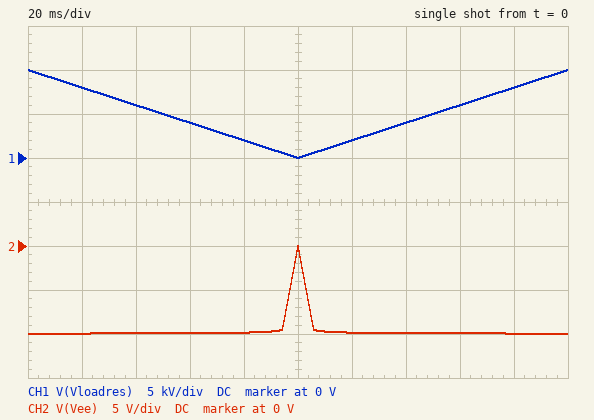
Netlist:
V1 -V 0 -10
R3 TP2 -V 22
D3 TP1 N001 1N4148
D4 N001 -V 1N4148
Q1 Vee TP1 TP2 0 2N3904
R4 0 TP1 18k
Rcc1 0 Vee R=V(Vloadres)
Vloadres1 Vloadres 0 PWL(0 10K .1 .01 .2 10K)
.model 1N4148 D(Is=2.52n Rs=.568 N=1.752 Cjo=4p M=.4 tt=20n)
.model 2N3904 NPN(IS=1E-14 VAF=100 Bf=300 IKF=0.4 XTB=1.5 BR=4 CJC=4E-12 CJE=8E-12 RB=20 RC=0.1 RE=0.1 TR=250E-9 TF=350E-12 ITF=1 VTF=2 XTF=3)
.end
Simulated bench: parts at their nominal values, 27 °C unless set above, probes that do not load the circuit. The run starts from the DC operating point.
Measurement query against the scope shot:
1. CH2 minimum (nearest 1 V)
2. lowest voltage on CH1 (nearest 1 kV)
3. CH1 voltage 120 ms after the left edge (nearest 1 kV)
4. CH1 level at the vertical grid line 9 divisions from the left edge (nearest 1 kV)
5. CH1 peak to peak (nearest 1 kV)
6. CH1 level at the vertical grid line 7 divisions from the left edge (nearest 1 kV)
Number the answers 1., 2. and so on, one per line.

1. -10 V
2. 0 V
3. 2 kV
4. 8 kV
5. 10 kV
6. 4 kV
